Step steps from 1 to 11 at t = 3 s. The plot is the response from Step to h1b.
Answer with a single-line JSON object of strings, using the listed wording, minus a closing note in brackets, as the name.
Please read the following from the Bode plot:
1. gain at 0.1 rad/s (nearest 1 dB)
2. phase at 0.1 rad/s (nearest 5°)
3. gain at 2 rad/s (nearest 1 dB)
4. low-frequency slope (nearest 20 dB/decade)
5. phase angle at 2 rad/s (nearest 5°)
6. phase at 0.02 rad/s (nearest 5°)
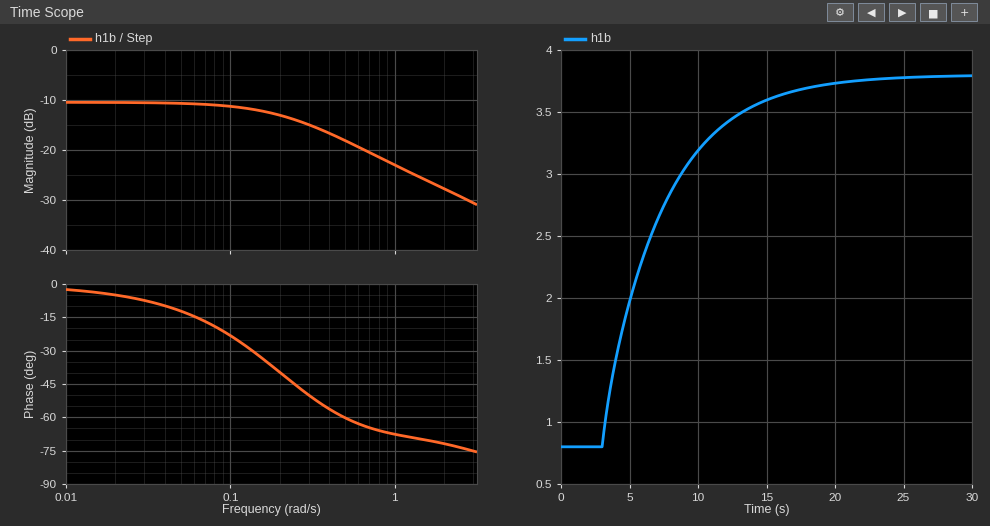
{"gain at 0.1 rad/s": "-11 dB", "phase at 0.1 rad/s": "-25°", "gain at 2 rad/s": "-28 dB", "low-frequency slope": "0 dB/decade", "phase angle at 2 rad/s": "-70°", "phase at 0.02 rad/s": "-5°"}
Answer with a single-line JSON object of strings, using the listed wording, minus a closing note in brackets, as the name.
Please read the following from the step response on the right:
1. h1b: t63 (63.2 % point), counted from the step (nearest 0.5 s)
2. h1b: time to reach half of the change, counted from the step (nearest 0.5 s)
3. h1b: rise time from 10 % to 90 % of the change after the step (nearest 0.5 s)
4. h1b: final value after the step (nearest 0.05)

{"h1b: t63 (63.2 % point), counted from the step": "4.5 s", "h1b: time to reach half of the change, counted from the step": "3.0 s", "h1b: rise time from 10 % to 90 % of the change after the step": "10.0 s", "h1b: final value after the step": "3.80"}
